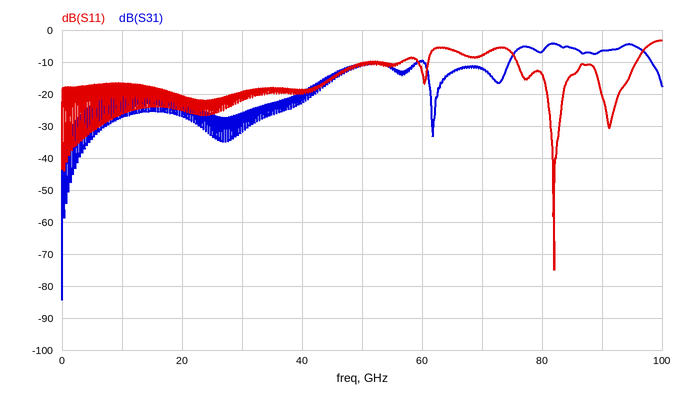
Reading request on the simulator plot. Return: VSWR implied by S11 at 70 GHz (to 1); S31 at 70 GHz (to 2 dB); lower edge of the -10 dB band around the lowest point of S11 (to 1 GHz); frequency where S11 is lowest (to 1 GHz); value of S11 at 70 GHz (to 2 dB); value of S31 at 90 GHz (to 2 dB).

2
-12 dB
76 GHz
82 GHz
-8 dB
-6 dB
